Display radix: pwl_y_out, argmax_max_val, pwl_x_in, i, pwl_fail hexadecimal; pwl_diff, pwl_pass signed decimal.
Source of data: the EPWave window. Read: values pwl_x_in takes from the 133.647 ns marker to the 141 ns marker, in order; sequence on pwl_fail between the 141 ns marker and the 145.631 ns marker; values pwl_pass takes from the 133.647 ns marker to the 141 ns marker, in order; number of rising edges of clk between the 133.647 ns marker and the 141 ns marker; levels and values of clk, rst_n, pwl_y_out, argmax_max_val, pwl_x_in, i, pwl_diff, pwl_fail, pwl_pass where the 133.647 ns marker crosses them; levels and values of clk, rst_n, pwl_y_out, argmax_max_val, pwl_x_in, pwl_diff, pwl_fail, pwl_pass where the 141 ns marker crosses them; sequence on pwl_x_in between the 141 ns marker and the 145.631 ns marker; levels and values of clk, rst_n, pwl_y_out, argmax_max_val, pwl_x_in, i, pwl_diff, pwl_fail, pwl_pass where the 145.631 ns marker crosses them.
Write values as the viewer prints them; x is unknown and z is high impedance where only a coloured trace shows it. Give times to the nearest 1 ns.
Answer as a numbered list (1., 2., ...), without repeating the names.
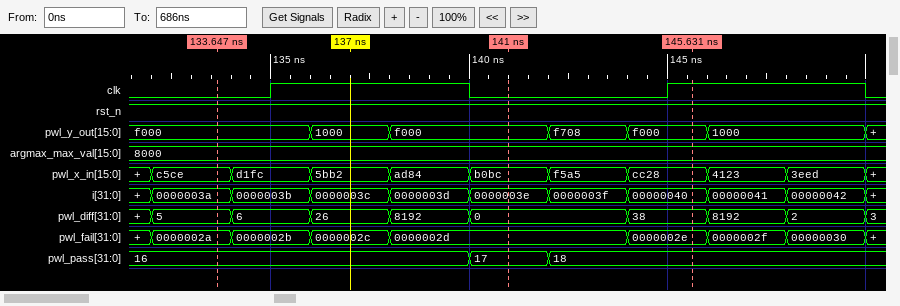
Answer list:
1. c5ce, d1fc, 5bb2, ad84, b0bc
2. 0000002d, 0000002e
3. 16, 17
4. 1
5. clk=0, rst_n=1, pwl_y_out=f000, argmax_max_val=8000, pwl_x_in=c5ce, i=0000003a, pwl_diff=5, pwl_fail=0000002a, pwl_pass=16
6. clk=0, rst_n=1, pwl_y_out=f000, argmax_max_val=8000, pwl_x_in=b0bc, pwl_diff=0, pwl_fail=0000002d, pwl_pass=17
7. b0bc, f5a5, cc28
8. clk=1, rst_n=1, pwl_y_out=f000, argmax_max_val=8000, pwl_x_in=cc28, i=00000040, pwl_diff=38, pwl_fail=0000002e, pwl_pass=18
